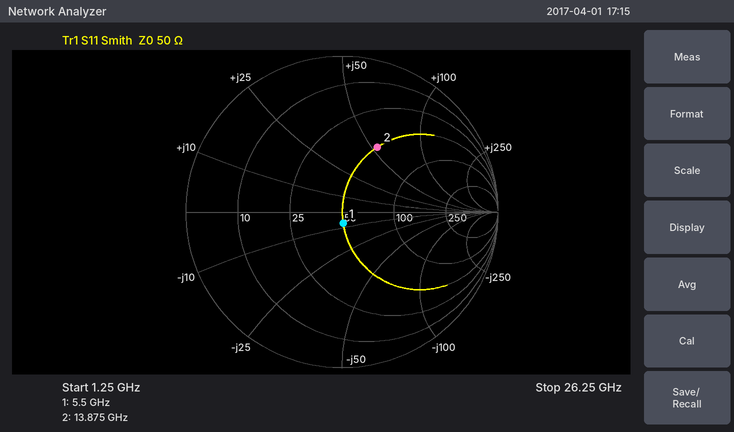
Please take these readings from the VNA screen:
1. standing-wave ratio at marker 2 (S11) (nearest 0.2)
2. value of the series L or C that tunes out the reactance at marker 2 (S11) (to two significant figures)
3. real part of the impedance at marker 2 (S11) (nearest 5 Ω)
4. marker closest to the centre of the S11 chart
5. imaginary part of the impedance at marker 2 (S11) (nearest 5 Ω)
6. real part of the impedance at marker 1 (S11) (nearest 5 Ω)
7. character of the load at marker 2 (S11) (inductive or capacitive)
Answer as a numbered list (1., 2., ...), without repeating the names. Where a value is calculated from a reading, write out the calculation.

1. 2.8
2. C = 1/(2π × 13.875 GHz × 55 Ω) ≈ 209 fF, so 210 fF to two significant figures
3. 50 Ω
4. marker 1
5. +55 Ω
6. 50 Ω
7. inductive
